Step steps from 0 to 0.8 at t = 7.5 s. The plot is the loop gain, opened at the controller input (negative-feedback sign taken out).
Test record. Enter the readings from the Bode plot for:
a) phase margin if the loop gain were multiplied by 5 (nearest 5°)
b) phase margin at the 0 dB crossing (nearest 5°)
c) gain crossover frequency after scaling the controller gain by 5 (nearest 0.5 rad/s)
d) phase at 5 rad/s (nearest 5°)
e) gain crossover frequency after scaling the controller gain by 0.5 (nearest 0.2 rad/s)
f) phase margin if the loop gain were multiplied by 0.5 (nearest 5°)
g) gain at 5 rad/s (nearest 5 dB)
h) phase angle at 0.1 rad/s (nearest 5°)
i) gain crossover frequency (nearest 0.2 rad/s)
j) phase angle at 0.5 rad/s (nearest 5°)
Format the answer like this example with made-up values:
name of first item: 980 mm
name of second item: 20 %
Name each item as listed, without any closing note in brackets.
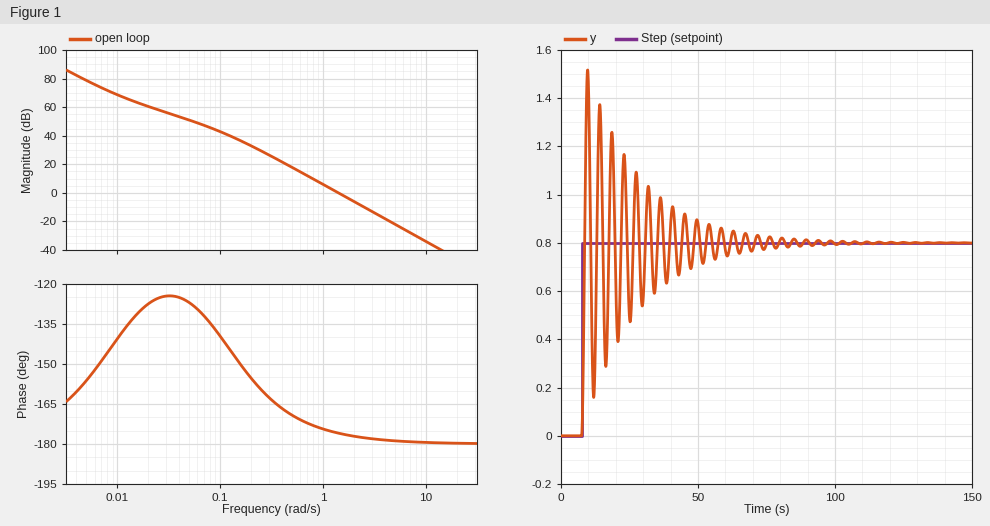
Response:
phase margin if the loop gain were multiplied by 5: 0°
phase margin at the 0 dB crossing: 5°
gain crossover frequency after scaling the controller gain by 5: 3.0 rad/s
phase at 5 rad/s: -180°
gain crossover frequency after scaling the controller gain by 0.5: 1.0 rad/s
phase margin if the loop gain were multiplied by 0.5: 5°
gain at 5 rad/s: -20 dB
phase angle at 0.1 rad/s: -140°
gain crossover frequency: 1.4 rad/s
phase angle at 0.5 rad/s: -170°
